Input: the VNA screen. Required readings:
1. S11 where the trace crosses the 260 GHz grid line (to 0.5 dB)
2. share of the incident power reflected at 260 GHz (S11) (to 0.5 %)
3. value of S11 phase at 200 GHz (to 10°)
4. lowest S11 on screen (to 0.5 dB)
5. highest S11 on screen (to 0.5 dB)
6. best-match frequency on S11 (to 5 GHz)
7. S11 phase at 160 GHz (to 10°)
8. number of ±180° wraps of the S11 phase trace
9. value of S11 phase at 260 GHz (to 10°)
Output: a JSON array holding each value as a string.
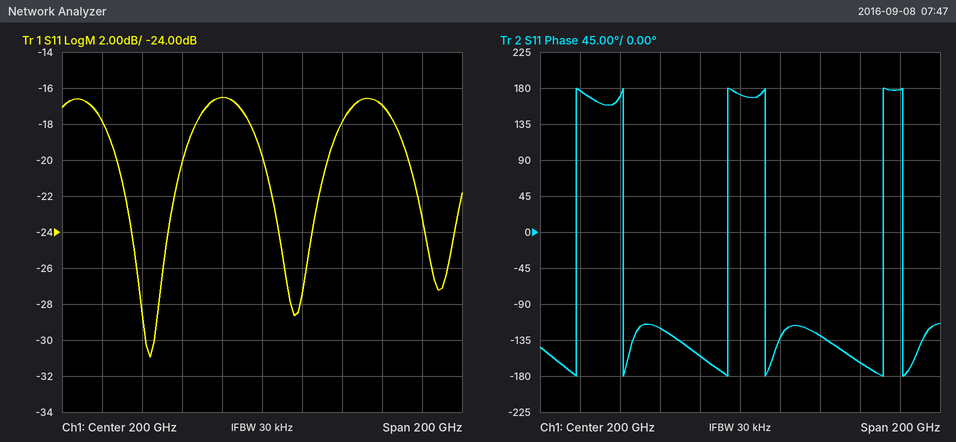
["-17.0 dB", "2.0 %", "170°", "-31.0 dB", "-16.5 dB", "145 GHz", "-120°", "6", "-160°"]
